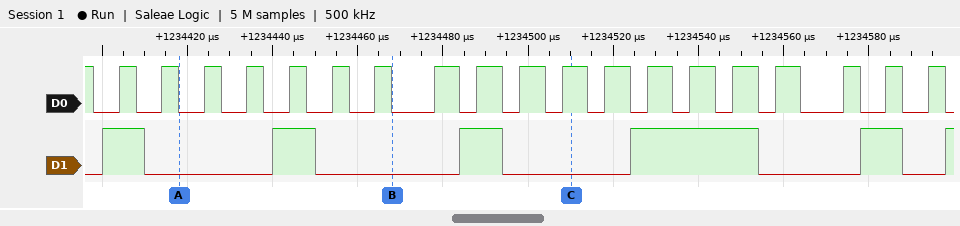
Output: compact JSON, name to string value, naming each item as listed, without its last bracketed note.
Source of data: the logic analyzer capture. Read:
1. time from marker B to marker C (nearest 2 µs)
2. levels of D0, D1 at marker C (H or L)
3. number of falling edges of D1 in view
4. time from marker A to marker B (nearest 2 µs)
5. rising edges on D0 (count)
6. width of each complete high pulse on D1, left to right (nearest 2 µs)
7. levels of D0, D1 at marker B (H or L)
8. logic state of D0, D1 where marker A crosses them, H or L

{"time from marker B to marker C": "42 µs", "levels of D0, D1 at marker C": "D0=H, D1=L", "number of falling edges of D1 in view": "5", "time from marker A to marker B": "50 µs", "rising edges on D0": "19", "width of each complete high pulse on D1, left to right": "10 µs, 10 µs, 10 µs, 30 µs, 10 µs", "levels of D0, D1 at marker B": "D0=L, D1=L", "logic state of D0, D1 where marker A crosses them, H or L": "D0=L, D1=L"}
